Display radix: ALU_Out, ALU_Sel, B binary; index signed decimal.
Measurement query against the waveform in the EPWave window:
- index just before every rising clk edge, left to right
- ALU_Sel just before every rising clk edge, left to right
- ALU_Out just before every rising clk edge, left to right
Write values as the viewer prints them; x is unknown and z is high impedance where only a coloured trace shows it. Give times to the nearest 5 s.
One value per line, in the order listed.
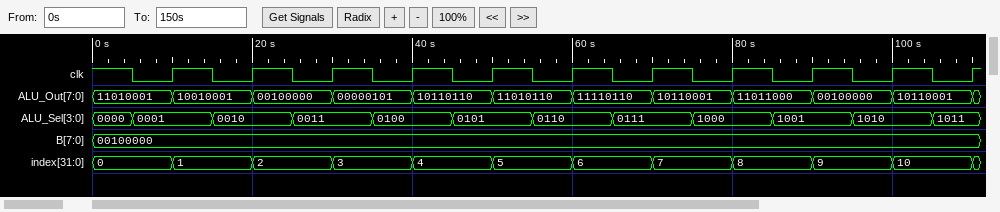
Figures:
0, 1, 2, 3, 4, 5, 6, 7, 8, 9, 10
0001, 0010, 0011, 0100, 0101, 0110, 0111, 1000, 1001, 1010, 1011
11010001, 10010001, 00100000, 00000101, 10110110, 11010110, 11110110, 10110001, 11011000, 00100000, 10110001
